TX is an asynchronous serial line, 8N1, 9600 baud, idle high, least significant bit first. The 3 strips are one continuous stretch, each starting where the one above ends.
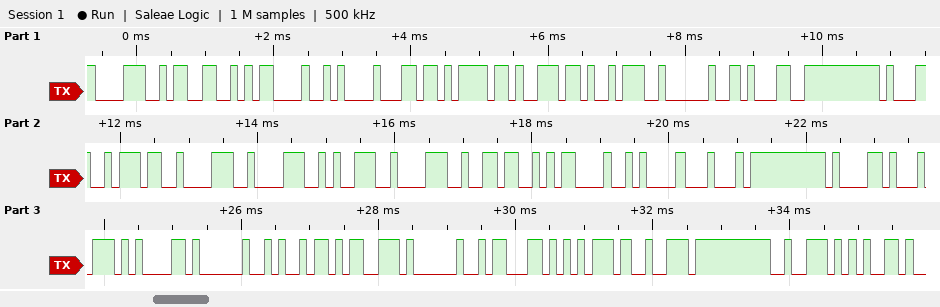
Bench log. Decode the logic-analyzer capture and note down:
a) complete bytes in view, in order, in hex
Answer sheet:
0x38 0x33 0x0D 0x0A 0x6C 0x6F 0x6E 0x3A 0x20 0x31 0x31 0x37 0x38 0x38 0x39 0x38 0x36 0x0D 0x0A 0x44 0x61 0x74 0x61 0x20 0x69 0x73 0x20 0x63 0x75 0x72 0x72 0x65
